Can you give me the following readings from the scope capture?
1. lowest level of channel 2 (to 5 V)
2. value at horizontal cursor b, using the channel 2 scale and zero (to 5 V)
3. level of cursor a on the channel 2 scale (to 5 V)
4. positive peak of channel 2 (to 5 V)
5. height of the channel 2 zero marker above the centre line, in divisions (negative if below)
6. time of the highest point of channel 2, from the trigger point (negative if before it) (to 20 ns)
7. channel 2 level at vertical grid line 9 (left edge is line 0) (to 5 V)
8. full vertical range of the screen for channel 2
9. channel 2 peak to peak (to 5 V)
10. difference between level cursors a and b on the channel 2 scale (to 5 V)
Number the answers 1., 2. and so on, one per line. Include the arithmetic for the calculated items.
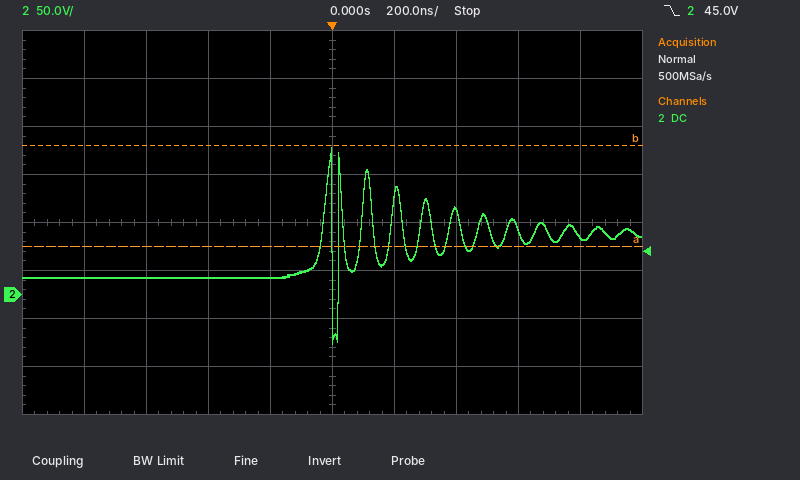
1. -50 V
2. 155 V
3. 50 V
4. 155 V
5. -1.5 div
6. 0 ns
7. 60 V
8. 400 V
9. 155 V − (-50 V) = 205 V
10. 105 V
